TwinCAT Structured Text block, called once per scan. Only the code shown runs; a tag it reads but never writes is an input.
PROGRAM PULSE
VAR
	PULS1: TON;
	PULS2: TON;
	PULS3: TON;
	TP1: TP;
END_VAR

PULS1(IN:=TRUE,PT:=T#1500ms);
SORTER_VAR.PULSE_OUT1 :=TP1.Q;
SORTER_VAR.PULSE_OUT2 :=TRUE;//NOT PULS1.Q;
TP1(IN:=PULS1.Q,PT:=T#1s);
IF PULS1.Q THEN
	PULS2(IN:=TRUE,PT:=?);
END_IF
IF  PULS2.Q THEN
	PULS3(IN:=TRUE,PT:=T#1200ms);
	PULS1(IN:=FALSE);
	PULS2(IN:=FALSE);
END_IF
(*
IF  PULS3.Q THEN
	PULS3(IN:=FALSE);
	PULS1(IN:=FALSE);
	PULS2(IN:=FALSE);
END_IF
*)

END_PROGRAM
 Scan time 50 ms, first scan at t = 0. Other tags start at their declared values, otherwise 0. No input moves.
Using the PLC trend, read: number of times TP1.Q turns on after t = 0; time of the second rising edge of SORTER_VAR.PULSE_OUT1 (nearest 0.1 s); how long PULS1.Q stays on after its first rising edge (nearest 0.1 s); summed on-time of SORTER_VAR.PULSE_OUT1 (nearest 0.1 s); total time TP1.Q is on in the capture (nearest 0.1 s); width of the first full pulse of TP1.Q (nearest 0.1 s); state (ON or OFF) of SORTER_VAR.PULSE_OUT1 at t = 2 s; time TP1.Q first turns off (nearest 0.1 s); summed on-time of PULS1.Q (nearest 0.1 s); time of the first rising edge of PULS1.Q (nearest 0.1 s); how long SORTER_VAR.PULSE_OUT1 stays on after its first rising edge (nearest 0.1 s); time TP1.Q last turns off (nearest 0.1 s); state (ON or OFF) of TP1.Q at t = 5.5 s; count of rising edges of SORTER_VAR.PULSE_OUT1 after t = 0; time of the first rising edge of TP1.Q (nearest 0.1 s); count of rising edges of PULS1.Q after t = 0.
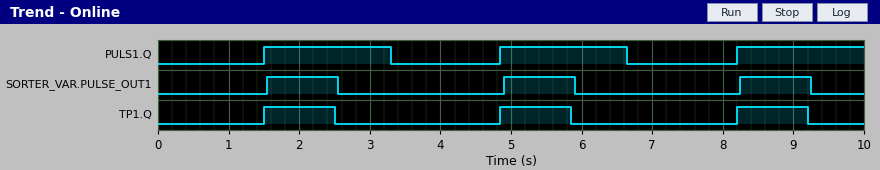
3
4.9 s
1.8 s
3.0 s
3.0 s
1.0 s
ON
2.5 s
5.4 s
1.5 s
1.0 s
9.2 s
ON
3
1.5 s
3
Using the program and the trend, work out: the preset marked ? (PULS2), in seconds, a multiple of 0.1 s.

1.8 s
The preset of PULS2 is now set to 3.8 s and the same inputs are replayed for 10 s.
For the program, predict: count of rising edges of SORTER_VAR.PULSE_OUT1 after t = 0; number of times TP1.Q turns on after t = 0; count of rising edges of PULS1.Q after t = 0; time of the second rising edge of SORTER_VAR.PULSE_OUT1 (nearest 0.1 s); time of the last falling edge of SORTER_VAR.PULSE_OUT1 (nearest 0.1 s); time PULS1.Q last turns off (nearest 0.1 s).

2
2
2
6.9 s
7.9 s
5.3 s
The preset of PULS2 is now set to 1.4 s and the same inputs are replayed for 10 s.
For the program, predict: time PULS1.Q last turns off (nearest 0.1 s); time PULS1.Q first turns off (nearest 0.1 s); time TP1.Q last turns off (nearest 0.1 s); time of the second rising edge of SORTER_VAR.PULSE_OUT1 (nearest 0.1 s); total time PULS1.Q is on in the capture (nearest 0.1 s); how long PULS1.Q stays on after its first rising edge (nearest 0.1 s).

8.8 s
2.9 s
8.4 s
4.5 s
4.2 s
1.4 s
